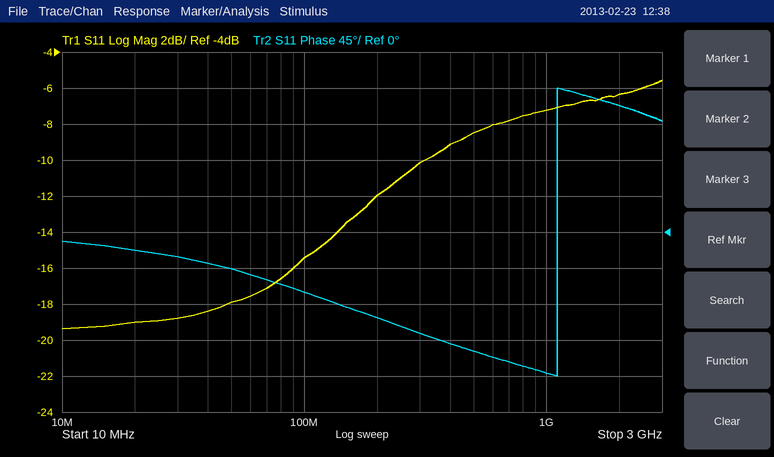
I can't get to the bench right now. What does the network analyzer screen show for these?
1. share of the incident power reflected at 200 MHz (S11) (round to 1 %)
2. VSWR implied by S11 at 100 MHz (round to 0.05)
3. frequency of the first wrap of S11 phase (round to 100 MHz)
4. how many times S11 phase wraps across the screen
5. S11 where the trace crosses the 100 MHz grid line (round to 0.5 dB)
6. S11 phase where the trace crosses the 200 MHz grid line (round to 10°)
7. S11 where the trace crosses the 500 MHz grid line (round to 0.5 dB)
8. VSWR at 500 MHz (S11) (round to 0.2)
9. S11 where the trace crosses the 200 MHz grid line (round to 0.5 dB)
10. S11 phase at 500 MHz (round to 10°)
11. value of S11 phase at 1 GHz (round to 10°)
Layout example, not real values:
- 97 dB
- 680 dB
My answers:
- 6 %
- 1.40
- 1.1 GHz
- 1
- -15.5 dB
- -110°
- -8.5 dB
- 2.2
- -12.0 dB
- -150°
- -180°
